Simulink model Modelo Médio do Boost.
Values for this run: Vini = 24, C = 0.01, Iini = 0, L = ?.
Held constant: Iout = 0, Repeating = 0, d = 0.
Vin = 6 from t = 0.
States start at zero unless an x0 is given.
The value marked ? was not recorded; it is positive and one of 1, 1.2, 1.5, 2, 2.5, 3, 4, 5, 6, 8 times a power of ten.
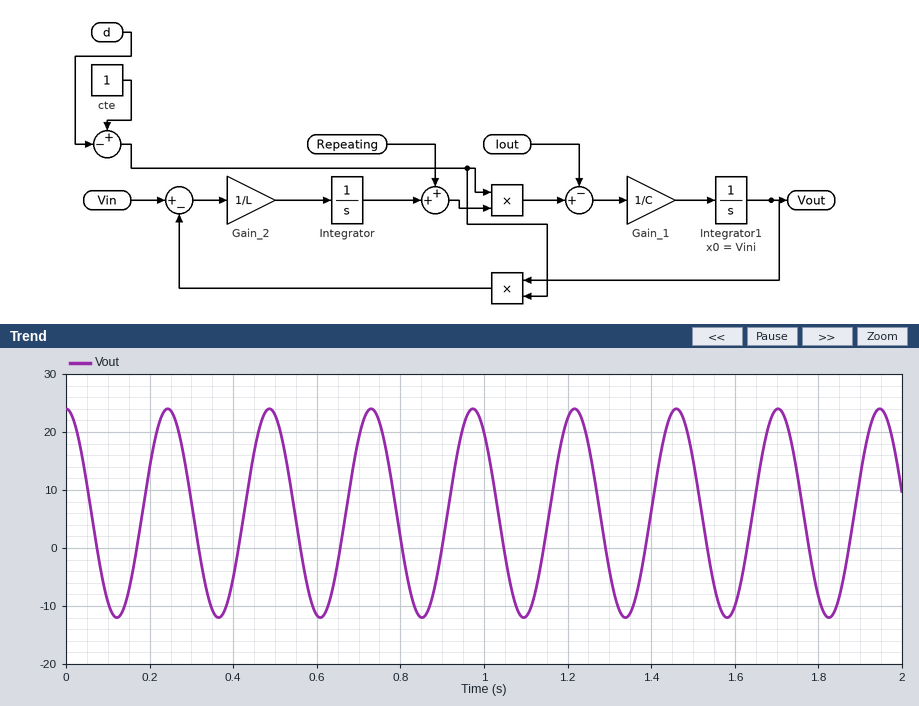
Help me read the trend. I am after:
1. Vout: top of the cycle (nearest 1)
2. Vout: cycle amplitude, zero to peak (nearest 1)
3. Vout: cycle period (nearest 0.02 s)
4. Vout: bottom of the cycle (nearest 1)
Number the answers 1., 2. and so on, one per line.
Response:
1. 24
2. 18
3. 0.24 s
4. -12
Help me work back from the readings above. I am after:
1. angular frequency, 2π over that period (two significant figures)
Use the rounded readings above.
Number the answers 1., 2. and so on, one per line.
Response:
1. 26 rad/s
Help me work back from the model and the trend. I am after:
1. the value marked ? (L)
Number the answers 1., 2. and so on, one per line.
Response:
1. 0.15
